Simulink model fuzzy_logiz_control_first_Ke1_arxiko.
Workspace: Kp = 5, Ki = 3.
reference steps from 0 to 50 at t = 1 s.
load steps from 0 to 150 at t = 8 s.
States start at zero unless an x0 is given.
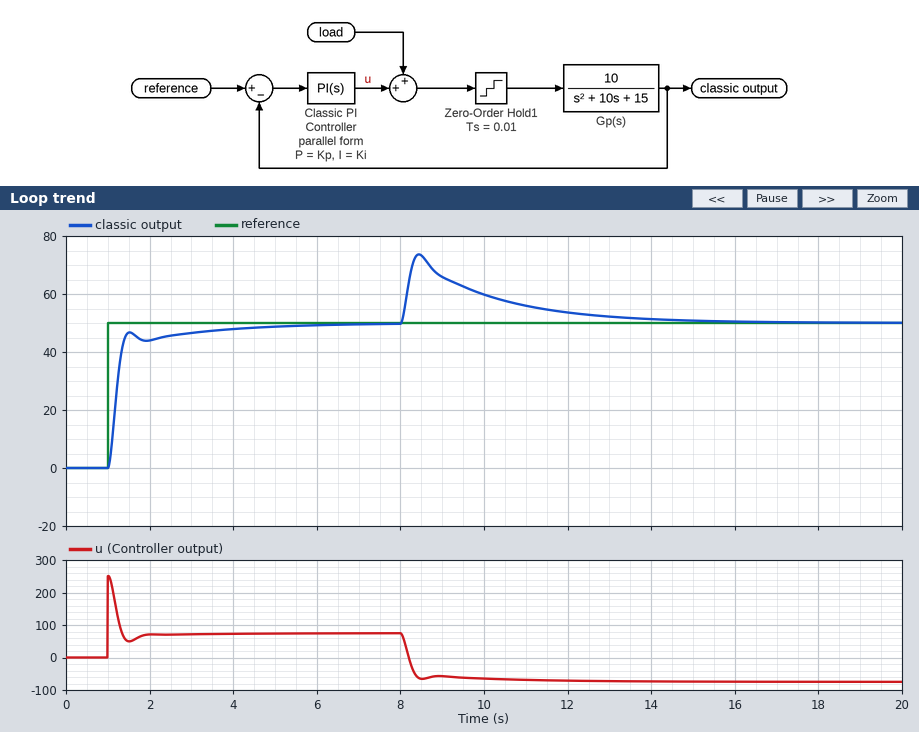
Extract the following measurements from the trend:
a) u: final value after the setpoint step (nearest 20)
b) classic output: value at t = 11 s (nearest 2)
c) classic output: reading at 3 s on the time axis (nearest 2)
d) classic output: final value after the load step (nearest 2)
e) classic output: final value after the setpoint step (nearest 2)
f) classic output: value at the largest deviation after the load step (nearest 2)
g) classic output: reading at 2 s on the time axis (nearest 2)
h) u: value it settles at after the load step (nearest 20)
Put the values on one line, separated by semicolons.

80; 56; 46; 50; 50; 74; 44; -80
